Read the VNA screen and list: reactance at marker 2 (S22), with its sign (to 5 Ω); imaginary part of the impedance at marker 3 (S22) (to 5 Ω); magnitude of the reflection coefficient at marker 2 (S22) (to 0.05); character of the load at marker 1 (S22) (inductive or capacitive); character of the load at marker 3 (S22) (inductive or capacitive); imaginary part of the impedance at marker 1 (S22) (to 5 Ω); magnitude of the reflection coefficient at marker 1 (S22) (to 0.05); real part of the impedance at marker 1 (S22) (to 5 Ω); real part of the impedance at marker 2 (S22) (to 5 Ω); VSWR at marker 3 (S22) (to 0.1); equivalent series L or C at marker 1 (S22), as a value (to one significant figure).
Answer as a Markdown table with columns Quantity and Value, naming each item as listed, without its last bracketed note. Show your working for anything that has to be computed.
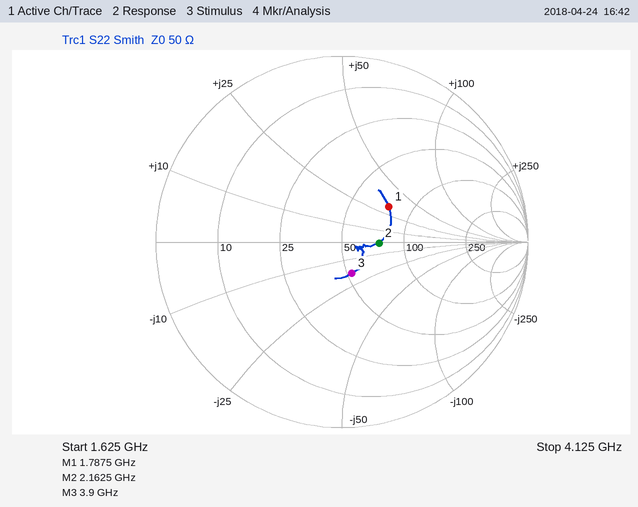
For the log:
| Quantity | Value |
|---|---|
| reactance at marker 2 (S22), with its sign | 0 Ω |
| imaginary part of the impedance at marker 3 (S22) | -20 Ω |
| magnitude of the reflection coefficient at marker 2 (S22) | 0.20 |
| character of the load at marker 1 (S22) | inductive |
| character of the load at marker 3 (S22) | capacitive |
| imaginary part of the impedance at marker 1 (S22) | +30 Ω |
| magnitude of the reflection coefficient at marker 1 (S22) | 0.30 |
| real part of the impedance at marker 1 (S22) | 75 Ω |
| real part of the impedance at marker 2 (S22) | 75 Ω |
| VSWR at marker 3 (S22) | 1.4 |
| equivalent series L or C at marker 1 (S22), as a value | L = 30 Ω/(2π × 1.7875 GHz) ≈ 3 nH |
